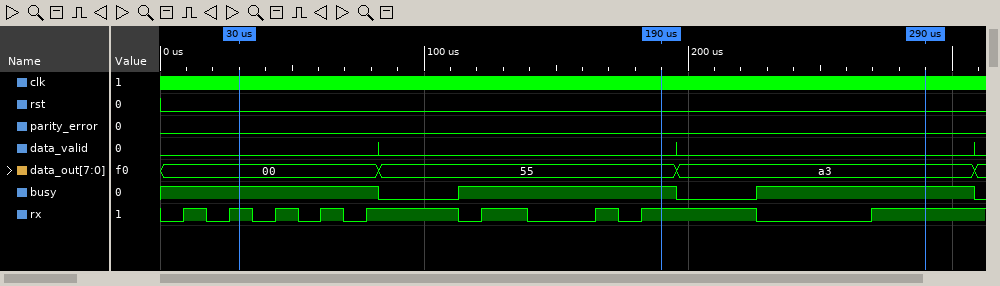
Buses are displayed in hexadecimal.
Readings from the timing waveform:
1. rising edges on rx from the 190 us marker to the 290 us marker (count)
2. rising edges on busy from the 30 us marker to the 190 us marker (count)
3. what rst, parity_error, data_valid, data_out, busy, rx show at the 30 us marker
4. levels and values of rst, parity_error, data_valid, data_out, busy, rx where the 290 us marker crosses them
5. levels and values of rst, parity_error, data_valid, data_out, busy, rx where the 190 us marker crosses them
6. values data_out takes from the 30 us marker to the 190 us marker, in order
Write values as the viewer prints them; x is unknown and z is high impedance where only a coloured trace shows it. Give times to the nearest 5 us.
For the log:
1
1
rst=0, parity_error=0, data_valid=0, data_out=00, busy=1, rx=1
rst=0, parity_error=0, data_valid=0, data_out=a3, busy=1, rx=1
rst=0, parity_error=0, data_valid=0, data_out=55, busy=1, rx=1
00, 55
